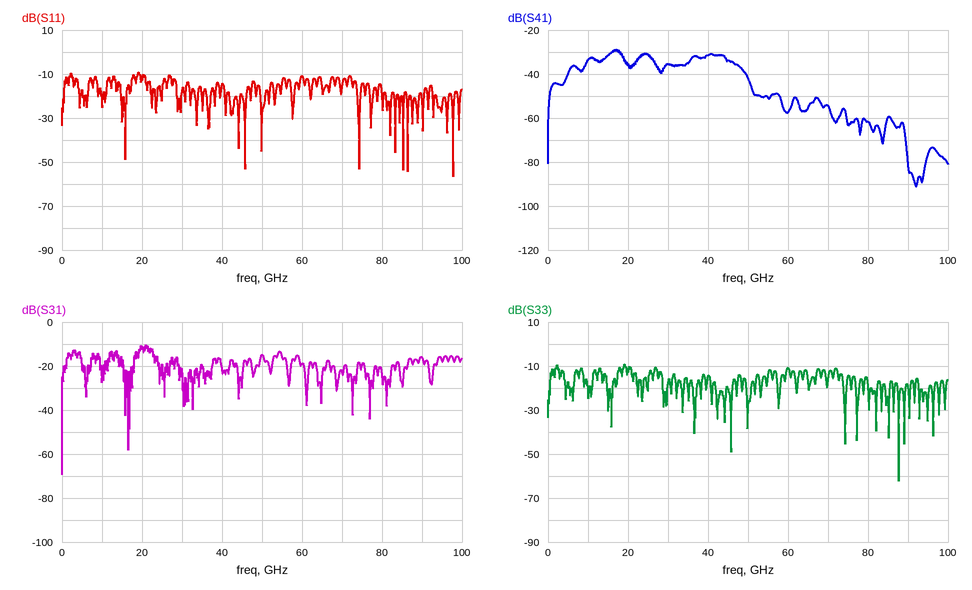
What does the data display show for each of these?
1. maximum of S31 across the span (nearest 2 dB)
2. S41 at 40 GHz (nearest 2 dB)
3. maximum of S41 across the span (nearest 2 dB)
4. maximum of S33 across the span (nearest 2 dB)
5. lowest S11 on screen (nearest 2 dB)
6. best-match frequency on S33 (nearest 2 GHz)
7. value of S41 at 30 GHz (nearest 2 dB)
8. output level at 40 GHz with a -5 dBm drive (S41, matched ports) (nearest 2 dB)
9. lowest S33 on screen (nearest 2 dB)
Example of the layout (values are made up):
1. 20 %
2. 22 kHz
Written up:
1. -10 dB
2. -32 dB
3. -28 dB
4. -10 dB
5. -56 dB
6. 88 GHz
7. -36 dB
8. -36 dBm
9. -62 dB
